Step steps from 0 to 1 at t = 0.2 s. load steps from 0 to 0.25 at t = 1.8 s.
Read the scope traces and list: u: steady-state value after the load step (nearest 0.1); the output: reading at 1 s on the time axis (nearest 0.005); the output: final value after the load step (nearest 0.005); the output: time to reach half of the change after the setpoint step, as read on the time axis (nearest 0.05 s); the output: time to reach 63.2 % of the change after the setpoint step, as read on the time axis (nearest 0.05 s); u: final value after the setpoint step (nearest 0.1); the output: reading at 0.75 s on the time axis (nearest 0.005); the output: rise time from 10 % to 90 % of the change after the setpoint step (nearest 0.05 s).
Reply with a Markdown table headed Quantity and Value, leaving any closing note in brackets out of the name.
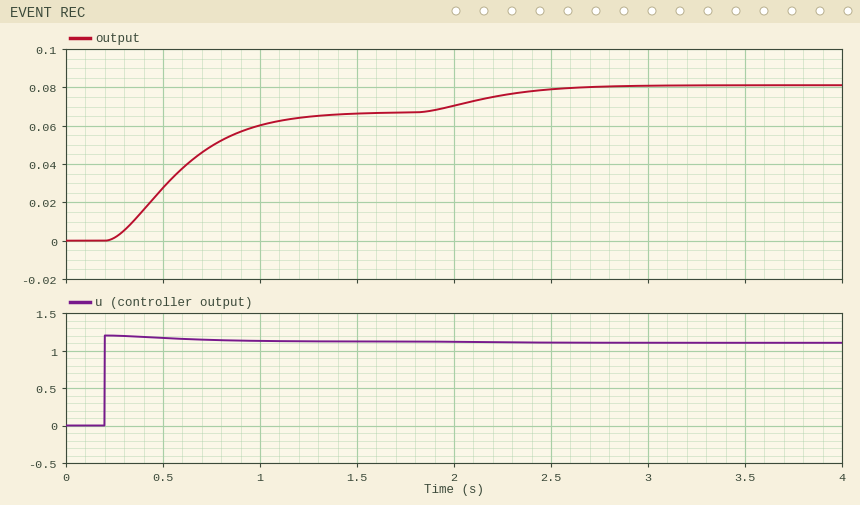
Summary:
| Quantity | Value |
|---|---|
| u: steady-state value after the load step | 1.1 |
| the output: reading at 1 s on the time axis | 0.060 |
| the output: final value after the load step | 0.080 |
| the output: time to reach half of the change after the setpoint step, as read on the time axis | 0.55 s |
| the output: time to reach 63.2 % of the change after the setpoint step, as read on the time axis | 0.65 s |
| u: final value after the setpoint step | 1.1 |
| the output: reading at 0.75 s on the time axis | 0.050 |
| the output: rise time from 10 % to 90 % of the change after the setpoint step | 0.70 s |
